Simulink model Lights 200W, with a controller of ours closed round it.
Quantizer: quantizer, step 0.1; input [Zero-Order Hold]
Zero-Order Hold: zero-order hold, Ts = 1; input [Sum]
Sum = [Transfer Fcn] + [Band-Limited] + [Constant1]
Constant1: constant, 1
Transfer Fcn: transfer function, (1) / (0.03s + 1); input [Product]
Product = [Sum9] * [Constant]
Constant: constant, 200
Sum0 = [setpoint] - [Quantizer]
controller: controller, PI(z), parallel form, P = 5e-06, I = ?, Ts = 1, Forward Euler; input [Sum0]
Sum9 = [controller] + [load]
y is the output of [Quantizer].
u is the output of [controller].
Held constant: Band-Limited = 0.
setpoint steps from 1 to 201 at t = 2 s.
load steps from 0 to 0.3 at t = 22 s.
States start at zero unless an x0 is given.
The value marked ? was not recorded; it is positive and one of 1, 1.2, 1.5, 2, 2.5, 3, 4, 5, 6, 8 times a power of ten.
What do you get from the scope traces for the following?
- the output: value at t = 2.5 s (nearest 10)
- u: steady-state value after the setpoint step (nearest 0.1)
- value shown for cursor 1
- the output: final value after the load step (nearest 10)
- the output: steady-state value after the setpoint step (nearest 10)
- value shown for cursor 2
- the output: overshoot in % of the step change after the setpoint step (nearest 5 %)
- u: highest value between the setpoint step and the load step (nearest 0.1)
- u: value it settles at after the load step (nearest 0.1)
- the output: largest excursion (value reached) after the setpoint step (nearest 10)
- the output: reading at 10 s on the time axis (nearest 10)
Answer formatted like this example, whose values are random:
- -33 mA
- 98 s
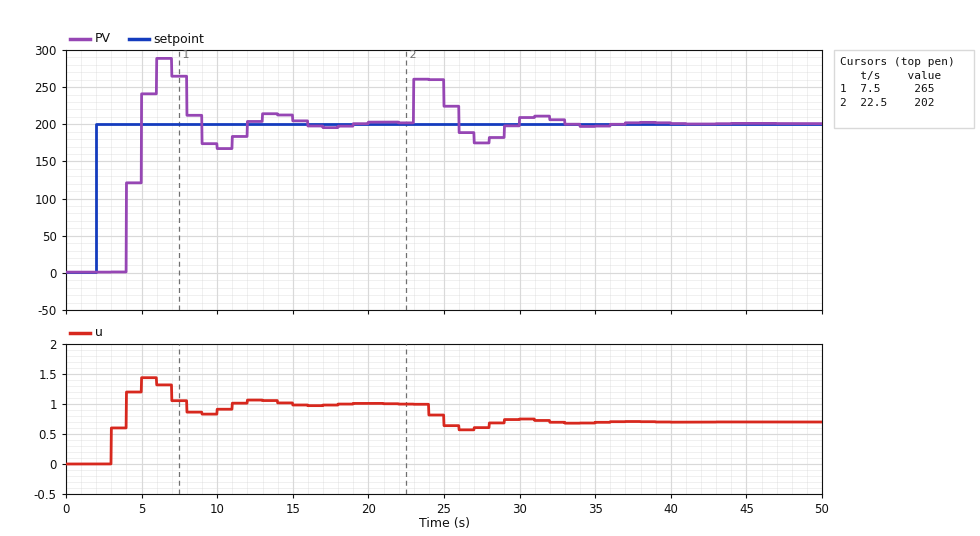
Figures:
- 0
- 1.0
- 265
- 200
- 200
- 202
- 45 %
- 1.4
- 0.7
- 290
- 170
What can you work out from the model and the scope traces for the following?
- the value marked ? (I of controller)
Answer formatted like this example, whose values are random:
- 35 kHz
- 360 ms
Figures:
- 0.003
